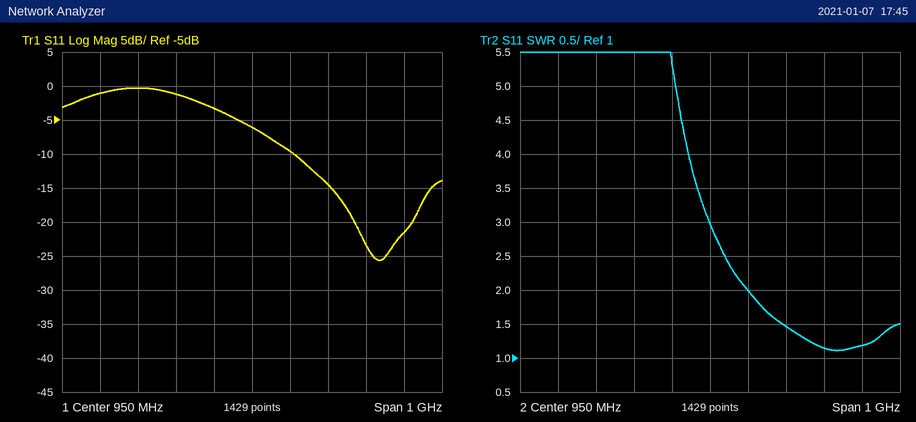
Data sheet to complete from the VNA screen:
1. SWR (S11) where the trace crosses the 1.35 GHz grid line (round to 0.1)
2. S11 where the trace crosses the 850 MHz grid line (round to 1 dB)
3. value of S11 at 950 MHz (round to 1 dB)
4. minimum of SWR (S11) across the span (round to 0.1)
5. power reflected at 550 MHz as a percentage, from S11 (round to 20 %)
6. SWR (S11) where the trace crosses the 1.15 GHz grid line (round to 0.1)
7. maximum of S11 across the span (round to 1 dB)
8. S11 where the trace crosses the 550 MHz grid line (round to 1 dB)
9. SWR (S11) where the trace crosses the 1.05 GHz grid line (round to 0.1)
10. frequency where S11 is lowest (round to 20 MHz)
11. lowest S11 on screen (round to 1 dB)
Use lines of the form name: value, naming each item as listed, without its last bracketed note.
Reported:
SWR (S11) where the trace crosses the 1.35 GHz grid line: 1.2
S11 where the trace crosses the 850 MHz grid line: -3 dB
value of S11 at 950 MHz: -6 dB
minimum of SWR (S11) across the span: 1.1
power reflected at 550 MHz as a percentage, from S11: 80 %
SWR (S11) where the trace crosses the 1.15 GHz grid line: 1.5
maximum of S11 across the span: 0 dB
S11 where the trace crosses the 550 MHz grid line: -1 dB
SWR (S11) where the trace crosses the 1.05 GHz grid line: 2.0
frequency where S11 is lowest: 1.28 GHz
lowest S11 on screen: -26 dB
